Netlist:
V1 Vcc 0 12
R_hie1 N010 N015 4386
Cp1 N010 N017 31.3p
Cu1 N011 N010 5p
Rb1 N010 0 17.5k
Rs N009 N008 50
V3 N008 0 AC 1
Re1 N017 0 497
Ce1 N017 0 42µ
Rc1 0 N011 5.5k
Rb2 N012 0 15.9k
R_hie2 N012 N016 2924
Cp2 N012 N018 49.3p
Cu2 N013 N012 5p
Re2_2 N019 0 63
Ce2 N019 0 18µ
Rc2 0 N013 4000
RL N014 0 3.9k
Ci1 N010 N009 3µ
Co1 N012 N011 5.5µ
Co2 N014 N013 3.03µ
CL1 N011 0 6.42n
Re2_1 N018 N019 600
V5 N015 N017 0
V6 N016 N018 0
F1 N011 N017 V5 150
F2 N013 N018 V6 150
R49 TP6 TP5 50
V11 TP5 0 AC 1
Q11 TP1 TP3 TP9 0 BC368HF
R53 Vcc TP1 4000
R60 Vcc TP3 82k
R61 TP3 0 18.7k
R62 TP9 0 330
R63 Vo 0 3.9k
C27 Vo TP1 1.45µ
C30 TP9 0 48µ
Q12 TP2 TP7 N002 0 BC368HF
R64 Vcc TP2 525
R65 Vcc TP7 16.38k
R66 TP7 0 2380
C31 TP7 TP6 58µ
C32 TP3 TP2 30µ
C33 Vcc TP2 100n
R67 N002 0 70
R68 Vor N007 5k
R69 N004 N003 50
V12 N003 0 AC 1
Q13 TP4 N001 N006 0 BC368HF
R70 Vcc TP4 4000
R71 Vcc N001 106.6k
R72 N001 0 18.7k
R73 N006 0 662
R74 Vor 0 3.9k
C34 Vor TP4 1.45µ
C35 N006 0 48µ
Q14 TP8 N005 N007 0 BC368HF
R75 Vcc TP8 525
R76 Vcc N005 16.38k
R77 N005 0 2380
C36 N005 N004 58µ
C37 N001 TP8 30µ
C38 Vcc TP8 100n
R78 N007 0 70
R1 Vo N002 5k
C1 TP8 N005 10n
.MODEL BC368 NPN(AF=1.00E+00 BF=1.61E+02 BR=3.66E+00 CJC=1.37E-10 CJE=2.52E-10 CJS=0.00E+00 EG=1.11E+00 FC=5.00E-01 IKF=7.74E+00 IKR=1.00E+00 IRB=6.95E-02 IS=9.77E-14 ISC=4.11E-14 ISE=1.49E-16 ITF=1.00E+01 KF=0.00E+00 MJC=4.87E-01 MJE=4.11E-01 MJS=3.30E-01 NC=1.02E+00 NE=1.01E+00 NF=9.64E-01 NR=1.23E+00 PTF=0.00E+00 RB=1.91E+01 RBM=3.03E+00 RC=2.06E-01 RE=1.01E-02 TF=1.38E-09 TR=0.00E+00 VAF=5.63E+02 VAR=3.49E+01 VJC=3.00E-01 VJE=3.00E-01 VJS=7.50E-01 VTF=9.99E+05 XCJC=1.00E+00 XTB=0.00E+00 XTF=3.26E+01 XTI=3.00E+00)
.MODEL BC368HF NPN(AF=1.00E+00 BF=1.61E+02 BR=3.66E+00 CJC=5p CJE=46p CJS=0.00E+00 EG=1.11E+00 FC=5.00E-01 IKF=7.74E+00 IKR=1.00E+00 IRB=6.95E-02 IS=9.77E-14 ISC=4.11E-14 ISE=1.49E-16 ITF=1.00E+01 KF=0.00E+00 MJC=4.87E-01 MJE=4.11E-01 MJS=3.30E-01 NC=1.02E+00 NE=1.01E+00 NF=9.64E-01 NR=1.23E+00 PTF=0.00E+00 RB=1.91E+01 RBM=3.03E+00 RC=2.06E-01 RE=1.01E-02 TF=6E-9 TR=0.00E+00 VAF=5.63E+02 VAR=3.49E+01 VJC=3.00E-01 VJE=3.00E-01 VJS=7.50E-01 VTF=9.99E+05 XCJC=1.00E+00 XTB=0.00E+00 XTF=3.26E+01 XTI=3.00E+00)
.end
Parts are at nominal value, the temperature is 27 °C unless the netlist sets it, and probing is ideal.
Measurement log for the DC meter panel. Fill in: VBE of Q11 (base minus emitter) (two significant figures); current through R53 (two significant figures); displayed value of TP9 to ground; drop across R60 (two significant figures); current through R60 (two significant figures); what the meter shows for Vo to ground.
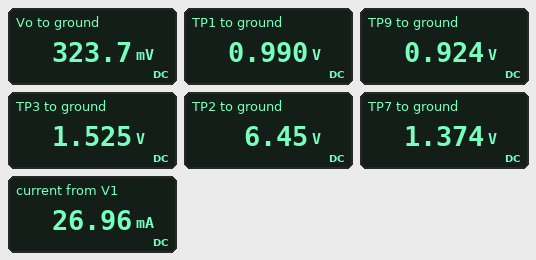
600 mV
2.8 mA
0.924 V
10 V
130 µA
323.7 mV
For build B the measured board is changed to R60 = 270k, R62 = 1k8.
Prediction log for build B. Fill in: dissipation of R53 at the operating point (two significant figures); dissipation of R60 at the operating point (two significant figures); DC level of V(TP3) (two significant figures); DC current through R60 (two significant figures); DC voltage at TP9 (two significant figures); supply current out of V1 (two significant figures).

69 µW
470 µW
760 mV
42 µA
240 mV
24 mA
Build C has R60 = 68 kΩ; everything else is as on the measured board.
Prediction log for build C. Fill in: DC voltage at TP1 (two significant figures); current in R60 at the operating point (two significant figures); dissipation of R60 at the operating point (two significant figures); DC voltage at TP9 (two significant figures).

980 mV
150 µA
1.6 mW
930 mV
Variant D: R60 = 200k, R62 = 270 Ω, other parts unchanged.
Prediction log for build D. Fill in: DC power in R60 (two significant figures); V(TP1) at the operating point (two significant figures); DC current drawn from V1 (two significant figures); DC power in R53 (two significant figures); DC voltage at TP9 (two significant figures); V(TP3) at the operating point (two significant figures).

620 µW
7.4 V
25 mA
5.3 mW
310 mV
890 mV
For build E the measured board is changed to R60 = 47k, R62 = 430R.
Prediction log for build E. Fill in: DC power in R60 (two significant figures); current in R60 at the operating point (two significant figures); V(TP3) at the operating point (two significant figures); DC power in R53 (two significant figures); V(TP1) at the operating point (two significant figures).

2.2 mW
220 µA
1.8 V
29 mW
1.2 V
